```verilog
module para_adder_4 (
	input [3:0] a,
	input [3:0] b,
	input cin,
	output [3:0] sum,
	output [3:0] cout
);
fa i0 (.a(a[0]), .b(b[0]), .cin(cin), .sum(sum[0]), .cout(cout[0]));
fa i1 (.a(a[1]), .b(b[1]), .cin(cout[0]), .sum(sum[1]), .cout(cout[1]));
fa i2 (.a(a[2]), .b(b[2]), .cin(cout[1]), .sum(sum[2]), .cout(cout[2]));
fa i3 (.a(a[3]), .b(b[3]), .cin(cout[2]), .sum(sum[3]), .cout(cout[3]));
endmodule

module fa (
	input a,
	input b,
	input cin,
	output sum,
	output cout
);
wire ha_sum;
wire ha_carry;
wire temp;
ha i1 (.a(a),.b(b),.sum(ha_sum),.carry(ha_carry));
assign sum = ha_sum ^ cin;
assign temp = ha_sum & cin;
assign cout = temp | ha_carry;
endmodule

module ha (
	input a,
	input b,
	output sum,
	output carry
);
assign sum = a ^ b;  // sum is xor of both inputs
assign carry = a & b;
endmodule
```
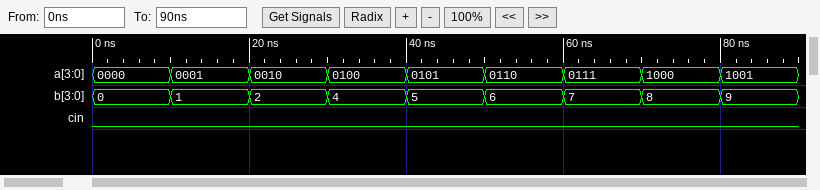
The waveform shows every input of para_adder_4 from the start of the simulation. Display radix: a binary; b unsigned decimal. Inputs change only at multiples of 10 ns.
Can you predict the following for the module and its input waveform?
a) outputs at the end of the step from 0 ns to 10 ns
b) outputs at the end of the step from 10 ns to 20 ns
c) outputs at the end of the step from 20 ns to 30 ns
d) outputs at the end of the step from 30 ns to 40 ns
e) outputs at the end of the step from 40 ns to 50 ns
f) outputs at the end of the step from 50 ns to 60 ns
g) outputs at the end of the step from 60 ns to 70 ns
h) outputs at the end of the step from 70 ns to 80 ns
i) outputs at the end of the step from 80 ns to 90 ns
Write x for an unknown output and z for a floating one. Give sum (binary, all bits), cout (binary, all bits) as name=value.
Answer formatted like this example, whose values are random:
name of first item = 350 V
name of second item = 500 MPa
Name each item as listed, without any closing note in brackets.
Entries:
outputs at the end of the step from 0 ns to 10 ns = sum=0000, cout=0000
outputs at the end of the step from 10 ns to 20 ns = sum=0010, cout=0001
outputs at the end of the step from 20 ns to 30 ns = sum=0100, cout=0010
outputs at the end of the step from 30 ns to 40 ns = sum=1000, cout=0100
outputs at the end of the step from 40 ns to 50 ns = sum=1010, cout=0101
outputs at the end of the step from 50 ns to 60 ns = sum=1100, cout=0110
outputs at the end of the step from 60 ns to 70 ns = sum=1110, cout=0111
outputs at the end of the step from 70 ns to 80 ns = sum=0000, cout=1000
outputs at the end of the step from 80 ns to 90 ns = sum=0010, cout=1001
